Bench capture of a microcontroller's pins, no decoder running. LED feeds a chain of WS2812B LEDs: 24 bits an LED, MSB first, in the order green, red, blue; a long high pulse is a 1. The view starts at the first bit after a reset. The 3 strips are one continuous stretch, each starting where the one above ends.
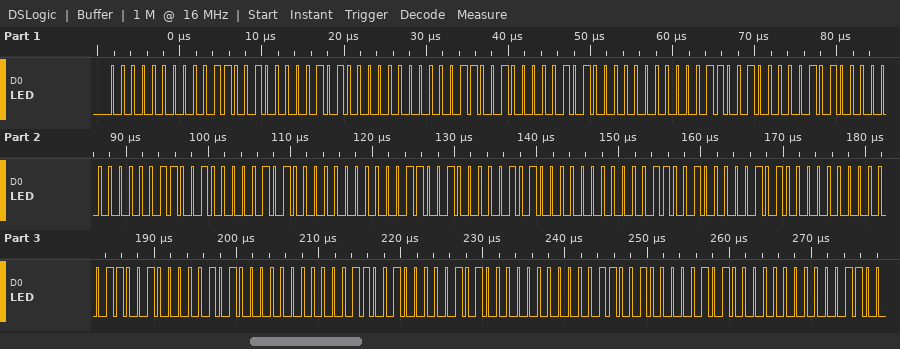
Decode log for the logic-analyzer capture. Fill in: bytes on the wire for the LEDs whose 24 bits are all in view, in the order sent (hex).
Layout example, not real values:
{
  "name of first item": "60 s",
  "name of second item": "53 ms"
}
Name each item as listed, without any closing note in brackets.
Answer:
{
  "bytes on the wire for the LEDs whose 24 bits are all in view, in the order sent": "00 32 0A 00 32 0A 00 32 0A 00 32 0A 00 32 0A 00 32 0A 00 32 0A 00 32 0A 00 32 0A"
}
